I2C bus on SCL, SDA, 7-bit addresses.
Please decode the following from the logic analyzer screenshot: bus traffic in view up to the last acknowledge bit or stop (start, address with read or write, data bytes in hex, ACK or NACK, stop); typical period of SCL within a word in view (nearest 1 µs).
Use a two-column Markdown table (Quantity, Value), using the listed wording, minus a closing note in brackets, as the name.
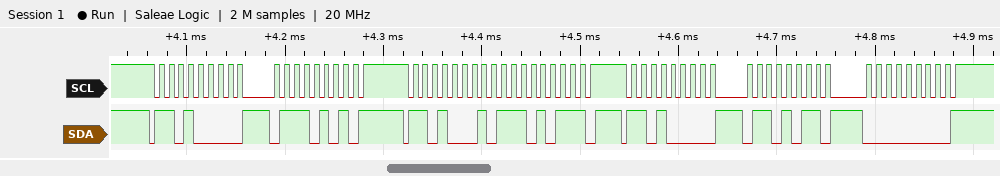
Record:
| Quantity | Value |
|---|---|
| bus traffic in view up to the last acknowledge bit or stop | start, address 68 write ACK, 75 ACK, repeated start, address 68 read ACK, EB NACK, stop, start, address 68 write ACK, 6B ACK, 00 ACK |
| typical period of SCL within a word in view | 10 µs |
